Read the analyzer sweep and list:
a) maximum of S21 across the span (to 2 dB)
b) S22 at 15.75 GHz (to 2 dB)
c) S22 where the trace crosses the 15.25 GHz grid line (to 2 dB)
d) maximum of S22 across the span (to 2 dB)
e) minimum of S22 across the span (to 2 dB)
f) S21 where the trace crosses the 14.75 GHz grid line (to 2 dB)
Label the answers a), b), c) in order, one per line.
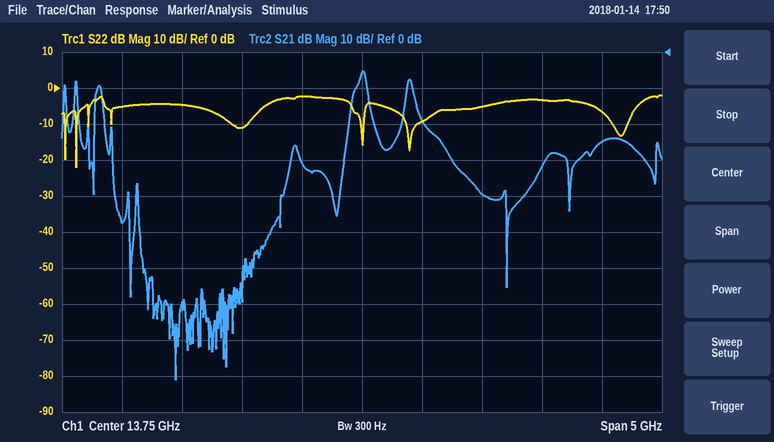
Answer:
a) -6 dB
b) -6 dB
c) -4 dB
d) -2 dB
e) -22 dB
f) -40 dB
